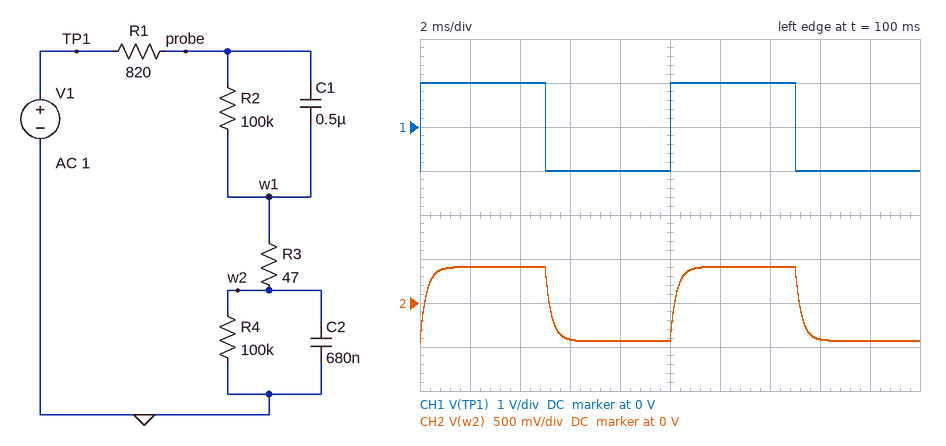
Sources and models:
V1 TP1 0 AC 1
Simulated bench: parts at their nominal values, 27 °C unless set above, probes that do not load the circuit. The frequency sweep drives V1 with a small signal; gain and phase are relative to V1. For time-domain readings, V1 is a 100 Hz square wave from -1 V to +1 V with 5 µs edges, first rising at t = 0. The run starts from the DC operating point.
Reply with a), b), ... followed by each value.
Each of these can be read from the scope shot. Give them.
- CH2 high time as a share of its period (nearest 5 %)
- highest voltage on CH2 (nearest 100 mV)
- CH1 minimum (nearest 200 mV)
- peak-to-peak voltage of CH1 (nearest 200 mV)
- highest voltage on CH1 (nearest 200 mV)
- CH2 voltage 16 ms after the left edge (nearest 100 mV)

a) 50 %
b) 400 mV
c) -1.0 V
d) 2.0 V
e) 1.0 V
f) -400 mV
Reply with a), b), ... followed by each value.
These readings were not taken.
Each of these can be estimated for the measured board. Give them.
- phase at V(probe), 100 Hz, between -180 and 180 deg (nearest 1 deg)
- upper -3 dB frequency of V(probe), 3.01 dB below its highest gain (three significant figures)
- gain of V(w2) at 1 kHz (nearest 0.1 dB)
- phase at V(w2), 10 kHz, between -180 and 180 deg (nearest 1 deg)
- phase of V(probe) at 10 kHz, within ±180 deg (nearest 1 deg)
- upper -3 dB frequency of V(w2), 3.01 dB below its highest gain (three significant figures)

a) -8 deg
b) 642 Hz
c) -12.9 dB
d) -86 deg
e) -46 deg
f) 423 Hz
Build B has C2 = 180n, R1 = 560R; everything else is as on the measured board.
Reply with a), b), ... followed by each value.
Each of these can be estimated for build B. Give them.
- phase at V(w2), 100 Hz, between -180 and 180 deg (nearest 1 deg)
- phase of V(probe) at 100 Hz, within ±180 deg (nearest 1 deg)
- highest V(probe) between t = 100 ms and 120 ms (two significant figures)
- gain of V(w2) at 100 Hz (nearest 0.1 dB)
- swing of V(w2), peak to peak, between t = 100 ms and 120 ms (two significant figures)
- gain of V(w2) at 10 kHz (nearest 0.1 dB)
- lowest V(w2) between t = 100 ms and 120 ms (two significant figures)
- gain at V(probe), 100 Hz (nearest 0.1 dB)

a) -2 deg
b) -3 deg
c) 1.0 V
d) -2.7 dB
e) 1.5 V
f) -16.9 dB
g) -740 mV
h) 0 dB
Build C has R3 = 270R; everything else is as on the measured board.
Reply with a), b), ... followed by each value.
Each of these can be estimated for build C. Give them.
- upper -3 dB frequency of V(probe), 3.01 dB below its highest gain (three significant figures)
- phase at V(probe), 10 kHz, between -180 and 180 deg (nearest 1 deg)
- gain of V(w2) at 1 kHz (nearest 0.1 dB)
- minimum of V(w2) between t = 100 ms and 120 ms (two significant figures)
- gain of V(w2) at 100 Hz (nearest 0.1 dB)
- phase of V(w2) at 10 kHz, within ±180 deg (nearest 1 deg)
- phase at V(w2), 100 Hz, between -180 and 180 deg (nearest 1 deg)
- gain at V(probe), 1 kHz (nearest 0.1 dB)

a) 544 Hz
b) -9 deg
c) -14.4 dB
d) -440 mV
e) -7.7 dB
f) -87 deg
g) -11 deg
h) -6.0 dB
